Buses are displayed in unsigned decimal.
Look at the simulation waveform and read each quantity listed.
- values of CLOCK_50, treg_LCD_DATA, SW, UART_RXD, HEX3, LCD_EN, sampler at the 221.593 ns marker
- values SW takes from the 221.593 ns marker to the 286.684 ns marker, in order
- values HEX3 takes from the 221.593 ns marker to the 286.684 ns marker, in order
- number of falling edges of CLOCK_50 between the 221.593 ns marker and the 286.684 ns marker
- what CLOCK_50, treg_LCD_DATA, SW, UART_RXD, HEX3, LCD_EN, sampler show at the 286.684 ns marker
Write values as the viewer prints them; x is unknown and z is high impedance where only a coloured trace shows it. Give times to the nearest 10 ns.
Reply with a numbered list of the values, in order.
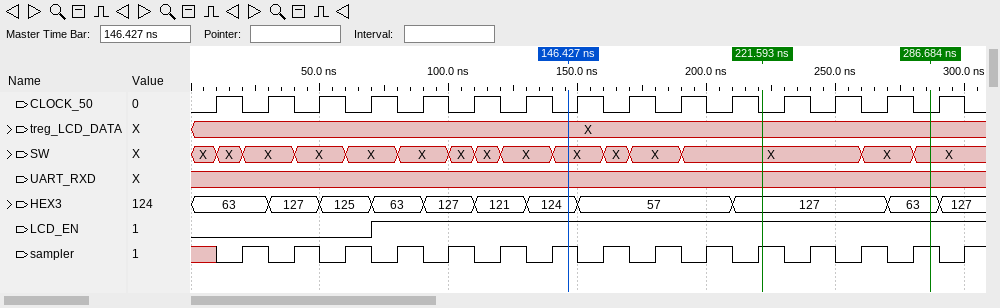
1. CLOCK_50=0, treg_LCD_DATA=X, SW=X, UART_RXD=x, HEX3=127, LCD_EN=1, sampler=1
2. X, X, X
3. 127, 63
4. 3
5. CLOCK_50=0, treg_LCD_DATA=X, SW=X, UART_RXD=x, HEX3=63, LCD_EN=1, sampler=1
